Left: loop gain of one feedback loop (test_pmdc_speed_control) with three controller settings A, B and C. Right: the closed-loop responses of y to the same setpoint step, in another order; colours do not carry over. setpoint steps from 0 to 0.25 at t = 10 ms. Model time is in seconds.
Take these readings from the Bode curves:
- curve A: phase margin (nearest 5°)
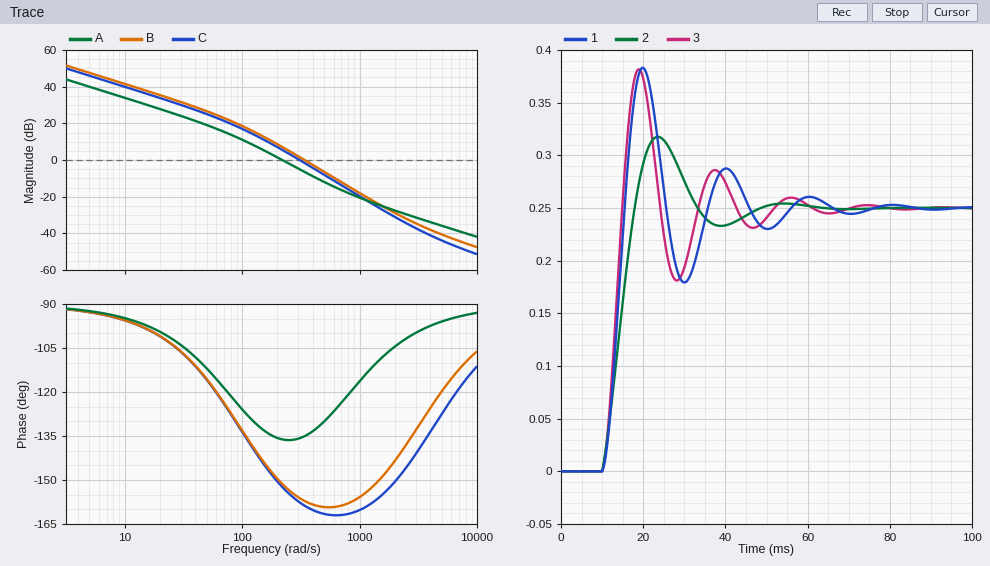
45°
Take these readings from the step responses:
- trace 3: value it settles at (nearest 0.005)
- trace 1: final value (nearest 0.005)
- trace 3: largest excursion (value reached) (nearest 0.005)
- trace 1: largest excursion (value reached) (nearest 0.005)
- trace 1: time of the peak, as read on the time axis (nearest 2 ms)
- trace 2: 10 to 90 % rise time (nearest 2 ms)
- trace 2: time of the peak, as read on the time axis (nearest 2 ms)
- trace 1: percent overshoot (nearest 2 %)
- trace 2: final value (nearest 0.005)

0.250
0.250
0.380
0.385
20 ms
6 ms
24 ms
54 %
0.250
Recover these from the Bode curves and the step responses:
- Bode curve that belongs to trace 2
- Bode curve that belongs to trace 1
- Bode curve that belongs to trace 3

A
C
B
